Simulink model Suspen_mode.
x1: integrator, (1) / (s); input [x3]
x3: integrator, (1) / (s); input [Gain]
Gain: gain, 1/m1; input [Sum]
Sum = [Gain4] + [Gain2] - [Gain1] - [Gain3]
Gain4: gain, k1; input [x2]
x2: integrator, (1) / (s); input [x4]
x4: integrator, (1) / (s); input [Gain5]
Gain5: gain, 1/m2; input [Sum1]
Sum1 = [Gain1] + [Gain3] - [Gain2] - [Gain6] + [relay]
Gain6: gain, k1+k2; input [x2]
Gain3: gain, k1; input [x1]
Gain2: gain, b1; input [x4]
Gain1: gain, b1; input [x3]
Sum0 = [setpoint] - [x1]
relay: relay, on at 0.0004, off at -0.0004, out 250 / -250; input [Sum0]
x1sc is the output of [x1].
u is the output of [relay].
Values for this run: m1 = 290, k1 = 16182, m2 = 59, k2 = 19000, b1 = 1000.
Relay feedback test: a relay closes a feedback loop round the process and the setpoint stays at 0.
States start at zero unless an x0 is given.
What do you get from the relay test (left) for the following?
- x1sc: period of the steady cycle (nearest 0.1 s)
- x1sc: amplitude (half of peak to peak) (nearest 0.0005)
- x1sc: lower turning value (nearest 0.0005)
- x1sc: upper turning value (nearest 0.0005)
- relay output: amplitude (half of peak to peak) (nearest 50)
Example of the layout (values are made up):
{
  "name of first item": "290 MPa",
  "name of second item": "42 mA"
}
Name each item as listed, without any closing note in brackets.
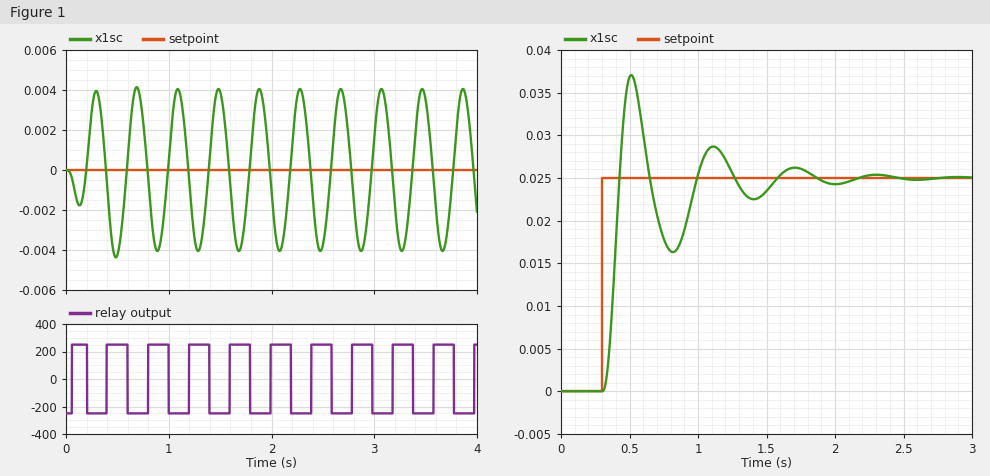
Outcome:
{
  "x1sc: period of the steady cycle": "0.4 s",
  "x1sc: amplitude (half of peak to peak)": "0.0040",
  "x1sc: lower turning value": "-0.0040",
  "x1sc: upper turning value": "0.0040",
  "relay output: amplitude (half of peak to peak)": "250"
}
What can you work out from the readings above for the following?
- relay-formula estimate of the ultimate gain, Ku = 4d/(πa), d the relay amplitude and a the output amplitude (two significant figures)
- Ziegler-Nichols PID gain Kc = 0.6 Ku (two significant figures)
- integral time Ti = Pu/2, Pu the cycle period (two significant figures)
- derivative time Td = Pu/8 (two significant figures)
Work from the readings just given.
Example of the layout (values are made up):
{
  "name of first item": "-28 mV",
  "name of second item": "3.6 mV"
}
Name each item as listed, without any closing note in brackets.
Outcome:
{
  "relay-formula estimate of the ultimate gain, Ku = 4d/(πa), d the relay amplitude and a the output amplitude": "80000",
  "Ziegler-Nichols PID gain Kc = 0.6 Ku": "48000",
  "integral time Ti = Pu/2, Pu the cycle period": "0.20 s",
  "derivative time Td = Pu/8": "0.050 s"
}
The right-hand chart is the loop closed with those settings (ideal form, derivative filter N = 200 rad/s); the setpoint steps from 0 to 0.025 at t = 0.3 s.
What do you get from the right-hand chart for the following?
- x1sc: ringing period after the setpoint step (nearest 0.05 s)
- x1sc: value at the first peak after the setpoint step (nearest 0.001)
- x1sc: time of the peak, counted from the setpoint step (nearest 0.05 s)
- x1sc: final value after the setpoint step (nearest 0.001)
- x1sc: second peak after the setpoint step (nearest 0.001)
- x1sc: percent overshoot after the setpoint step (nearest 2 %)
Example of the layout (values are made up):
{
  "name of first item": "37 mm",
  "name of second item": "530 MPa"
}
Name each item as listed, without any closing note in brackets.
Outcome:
{
  "x1sc: ringing period after the setpoint step": "0.60 s",
  "x1sc: value at the first peak after the setpoint step": "0.037",
  "x1sc: time of the peak, counted from the setpoint step": "0.20 s",
  "x1sc: final value after the setpoint step": "0.025",
  "x1sc: second peak after the setpoint step": "0.029",
  "x1sc: percent overshoot after the setpoint step": "48 %"
}
